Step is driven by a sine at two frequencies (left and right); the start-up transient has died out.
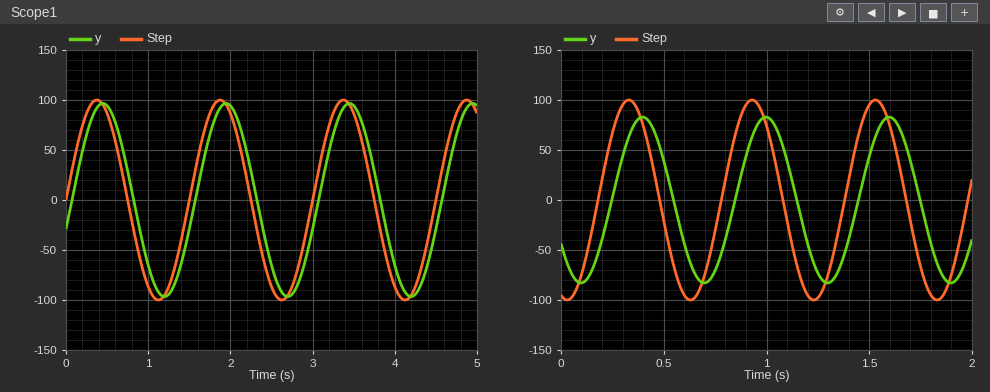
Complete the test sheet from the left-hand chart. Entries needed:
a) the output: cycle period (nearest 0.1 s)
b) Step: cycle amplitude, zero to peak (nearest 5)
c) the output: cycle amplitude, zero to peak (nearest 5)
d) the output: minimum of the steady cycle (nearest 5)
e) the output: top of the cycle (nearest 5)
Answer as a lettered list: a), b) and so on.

a) 1.5 s
b) 100
c) 95
d) -95
e) 95
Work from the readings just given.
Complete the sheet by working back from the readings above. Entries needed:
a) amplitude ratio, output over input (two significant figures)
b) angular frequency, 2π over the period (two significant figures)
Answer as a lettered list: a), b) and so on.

a) 0.95
b) 4.2 rad/s
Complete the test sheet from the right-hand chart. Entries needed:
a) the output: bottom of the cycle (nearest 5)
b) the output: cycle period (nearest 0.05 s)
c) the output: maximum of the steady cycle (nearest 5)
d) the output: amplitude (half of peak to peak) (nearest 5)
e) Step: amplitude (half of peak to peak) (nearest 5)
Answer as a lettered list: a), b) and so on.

a) -85
b) 0.60 s
c) 85
d) 85
e) 100
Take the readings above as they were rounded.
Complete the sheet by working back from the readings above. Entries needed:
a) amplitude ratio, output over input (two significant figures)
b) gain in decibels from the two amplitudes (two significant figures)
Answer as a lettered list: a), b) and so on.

a) 0.85
b) -1.4 dB
